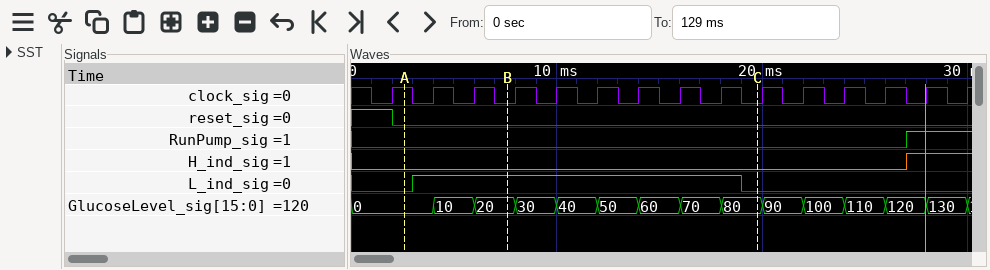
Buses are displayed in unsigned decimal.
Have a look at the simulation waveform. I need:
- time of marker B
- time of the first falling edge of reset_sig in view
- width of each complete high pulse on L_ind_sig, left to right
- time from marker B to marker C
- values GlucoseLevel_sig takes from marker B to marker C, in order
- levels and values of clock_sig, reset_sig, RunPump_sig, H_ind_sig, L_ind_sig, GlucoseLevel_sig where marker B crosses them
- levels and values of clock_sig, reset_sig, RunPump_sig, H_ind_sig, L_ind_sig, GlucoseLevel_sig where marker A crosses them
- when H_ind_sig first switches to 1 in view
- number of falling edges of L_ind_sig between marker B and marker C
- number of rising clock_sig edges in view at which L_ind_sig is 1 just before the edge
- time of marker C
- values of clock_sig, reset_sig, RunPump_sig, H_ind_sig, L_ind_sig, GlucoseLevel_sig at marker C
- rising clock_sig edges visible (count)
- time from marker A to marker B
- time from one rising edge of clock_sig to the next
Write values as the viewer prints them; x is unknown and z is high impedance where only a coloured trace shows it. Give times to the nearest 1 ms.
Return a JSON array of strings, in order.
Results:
["8 ms", "2 ms", "16 ms", "12 ms", "20, 30, 40, 50, 60, 70, 80", "clock_sig=0, reset_sig=0, RunPump_sig=0, H_ind_sig=0, L_ind_sig=1, GlucoseLevel_sig=20", "clock_sig=1, reset_sig=0, RunPump_sig=0, H_ind_sig=0, L_ind_sig=0, GlucoseLevel_sig=0", "27 ms", "1", "8", "20 ms", "clock_sig=0, reset_sig=0, RunPump_sig=0, H_ind_sig=0, L_ind_sig=0, GlucoseLevel_sig=80", "15", "5 ms", "2 ms"]
